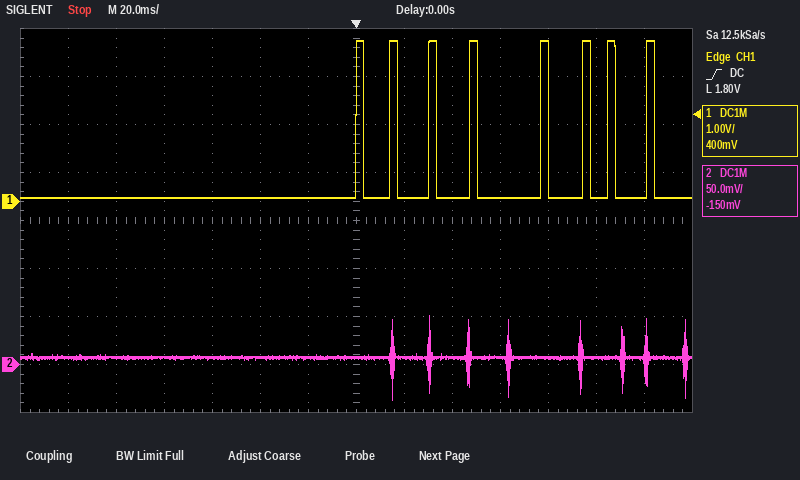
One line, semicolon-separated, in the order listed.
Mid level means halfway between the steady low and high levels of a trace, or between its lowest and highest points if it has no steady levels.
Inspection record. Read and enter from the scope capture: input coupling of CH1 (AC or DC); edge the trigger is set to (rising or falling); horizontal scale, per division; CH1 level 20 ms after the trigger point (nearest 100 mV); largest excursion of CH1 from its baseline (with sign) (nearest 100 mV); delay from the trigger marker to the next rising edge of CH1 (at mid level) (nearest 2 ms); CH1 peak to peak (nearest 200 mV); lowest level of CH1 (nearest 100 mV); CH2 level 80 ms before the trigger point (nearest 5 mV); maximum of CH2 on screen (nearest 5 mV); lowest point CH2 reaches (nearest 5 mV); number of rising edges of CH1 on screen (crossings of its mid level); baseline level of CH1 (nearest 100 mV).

DC; rising; 20 ms; 100 mV; +3.3 V; 14 ms; 3.2 V; 100 mV; 10 mV; 50 mV; -35 mV; 8; 100 mV
